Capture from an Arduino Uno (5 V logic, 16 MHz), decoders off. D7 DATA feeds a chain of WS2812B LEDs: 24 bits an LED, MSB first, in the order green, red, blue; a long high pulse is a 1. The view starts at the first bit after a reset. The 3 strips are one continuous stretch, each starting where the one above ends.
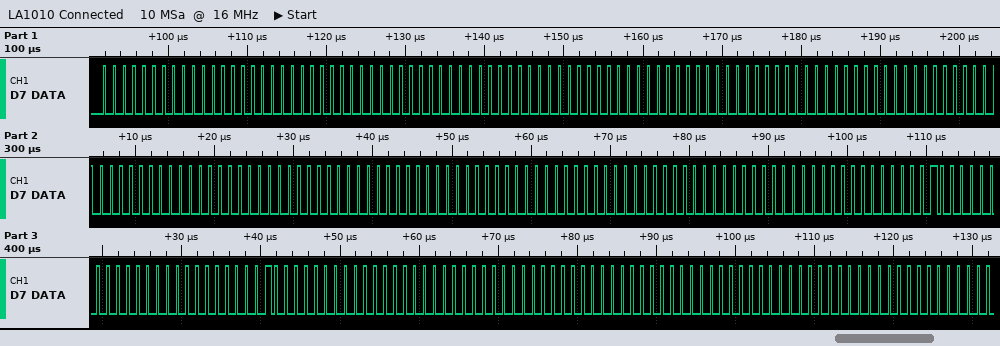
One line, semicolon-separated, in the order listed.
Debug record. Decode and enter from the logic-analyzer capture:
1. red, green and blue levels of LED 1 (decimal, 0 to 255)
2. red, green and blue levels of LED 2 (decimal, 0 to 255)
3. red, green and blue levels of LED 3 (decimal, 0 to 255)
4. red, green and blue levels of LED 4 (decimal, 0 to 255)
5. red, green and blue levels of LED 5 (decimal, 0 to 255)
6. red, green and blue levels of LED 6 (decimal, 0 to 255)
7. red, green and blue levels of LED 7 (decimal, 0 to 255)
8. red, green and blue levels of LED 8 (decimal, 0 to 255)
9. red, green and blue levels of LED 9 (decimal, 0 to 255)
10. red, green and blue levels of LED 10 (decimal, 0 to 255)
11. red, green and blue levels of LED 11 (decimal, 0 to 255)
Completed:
0, 0, 0; 0, 0, 0; 0, 0, 0; 0, 0, 0; 0, 0, 0; 0, 0, 0; 0, 0, 0; 0, 1, 0; 0, 1, 0; 0, 0, 0; 0, 0, 0
